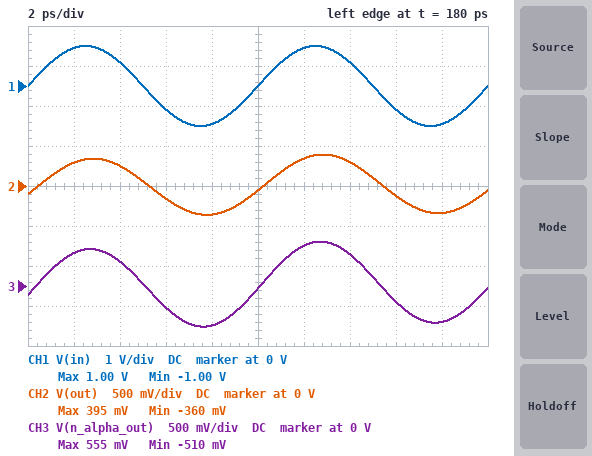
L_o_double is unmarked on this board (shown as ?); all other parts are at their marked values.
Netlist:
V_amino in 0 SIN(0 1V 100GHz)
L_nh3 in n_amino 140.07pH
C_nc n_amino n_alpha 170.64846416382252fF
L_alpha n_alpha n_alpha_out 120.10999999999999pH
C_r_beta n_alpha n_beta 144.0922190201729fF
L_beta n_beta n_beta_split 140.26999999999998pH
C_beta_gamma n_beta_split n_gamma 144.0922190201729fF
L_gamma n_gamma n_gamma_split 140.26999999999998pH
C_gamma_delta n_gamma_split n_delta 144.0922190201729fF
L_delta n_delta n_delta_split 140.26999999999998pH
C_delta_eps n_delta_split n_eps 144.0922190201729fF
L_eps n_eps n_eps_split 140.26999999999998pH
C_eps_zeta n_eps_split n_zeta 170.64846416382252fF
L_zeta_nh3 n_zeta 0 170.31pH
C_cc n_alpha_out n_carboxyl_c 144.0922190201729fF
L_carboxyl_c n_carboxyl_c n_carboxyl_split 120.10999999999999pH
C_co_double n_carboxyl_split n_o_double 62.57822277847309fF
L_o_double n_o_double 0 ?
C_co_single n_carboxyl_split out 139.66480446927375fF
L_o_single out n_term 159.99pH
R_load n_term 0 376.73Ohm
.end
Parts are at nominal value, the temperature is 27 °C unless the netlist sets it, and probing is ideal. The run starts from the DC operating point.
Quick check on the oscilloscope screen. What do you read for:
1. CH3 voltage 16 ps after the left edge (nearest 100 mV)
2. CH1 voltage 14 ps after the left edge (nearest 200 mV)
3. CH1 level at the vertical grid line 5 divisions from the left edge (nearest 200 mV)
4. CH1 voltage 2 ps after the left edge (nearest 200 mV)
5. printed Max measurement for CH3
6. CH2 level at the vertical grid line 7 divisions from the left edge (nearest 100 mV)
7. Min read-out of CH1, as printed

-200 mV
600 mV
0 V
1.0 V
555 mV
300 mV
-1.00 V
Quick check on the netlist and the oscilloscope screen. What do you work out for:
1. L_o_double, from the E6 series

330 pH
